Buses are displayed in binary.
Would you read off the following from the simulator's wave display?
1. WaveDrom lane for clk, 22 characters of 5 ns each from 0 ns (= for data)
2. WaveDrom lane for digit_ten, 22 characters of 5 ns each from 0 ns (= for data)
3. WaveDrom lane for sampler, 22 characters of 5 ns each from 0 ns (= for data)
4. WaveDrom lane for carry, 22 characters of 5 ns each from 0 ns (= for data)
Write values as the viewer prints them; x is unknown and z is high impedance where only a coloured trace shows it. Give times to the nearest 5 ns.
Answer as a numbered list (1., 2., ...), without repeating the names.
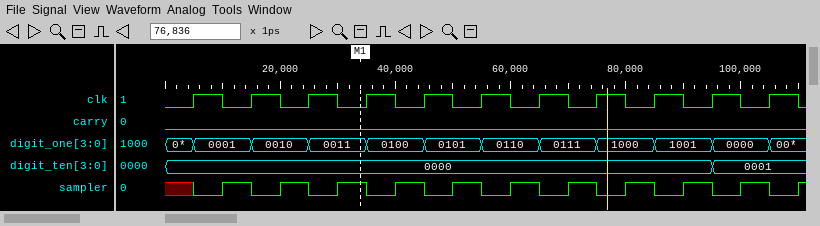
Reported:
1. {name: 'clk', wave: '0101010101010101010101'}
2. {name: 'digit_ten', wave: '=..................=..', data: '0000 0001'}
3. {name: 'sampler', wave: 'x010101010101010101010'}
4. {name: 'carry', wave: '0.....................'}
